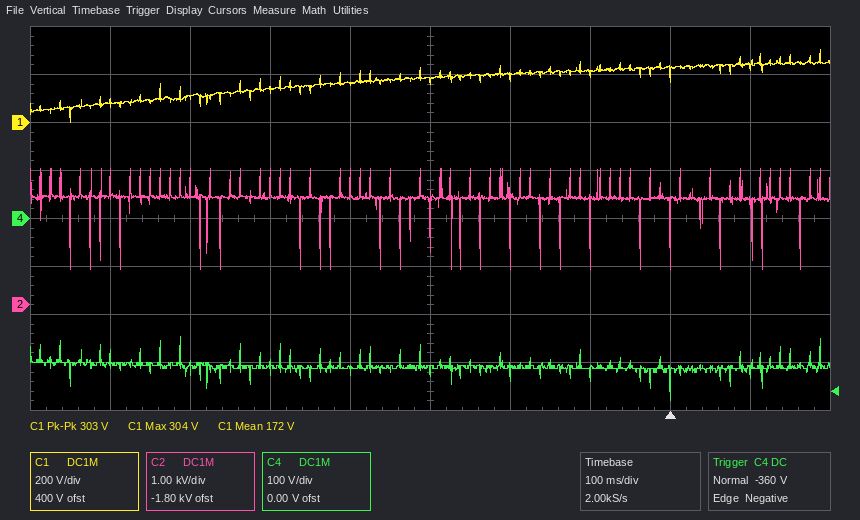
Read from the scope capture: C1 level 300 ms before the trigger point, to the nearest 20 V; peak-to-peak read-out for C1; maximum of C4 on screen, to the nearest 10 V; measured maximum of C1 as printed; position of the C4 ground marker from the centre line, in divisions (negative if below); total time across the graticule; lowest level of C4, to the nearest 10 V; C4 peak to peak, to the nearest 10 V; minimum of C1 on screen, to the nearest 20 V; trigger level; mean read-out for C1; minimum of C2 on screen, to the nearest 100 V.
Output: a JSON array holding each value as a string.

["180 V", "303 V", "-250 V", "304 V", "0.0 div", "1 s", "-380 V", "130 V", "0 V", "-360 V", "172 V", "700 V"]
